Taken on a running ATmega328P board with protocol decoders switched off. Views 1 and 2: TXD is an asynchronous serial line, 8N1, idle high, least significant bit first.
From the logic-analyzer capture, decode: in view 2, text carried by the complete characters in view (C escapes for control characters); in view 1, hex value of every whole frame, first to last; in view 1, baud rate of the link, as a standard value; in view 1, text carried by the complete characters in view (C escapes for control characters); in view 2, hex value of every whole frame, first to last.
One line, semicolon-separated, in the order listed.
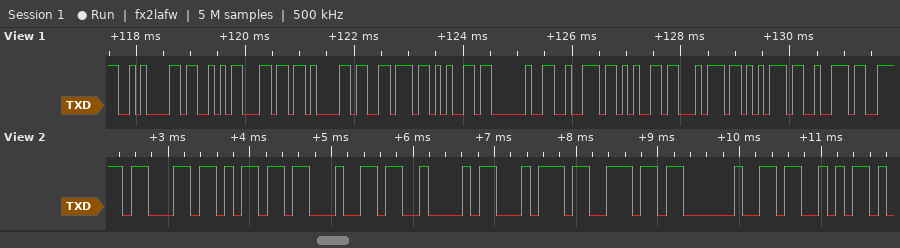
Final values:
"cmdBtn S"; 0A 53 6C 61 76 65 20 72 65 74 75 72; 9600 baud; "\nSlave retur"; 0x63 0x6D 0x64 0x42 0x74 0x6E 0x20 0x53
